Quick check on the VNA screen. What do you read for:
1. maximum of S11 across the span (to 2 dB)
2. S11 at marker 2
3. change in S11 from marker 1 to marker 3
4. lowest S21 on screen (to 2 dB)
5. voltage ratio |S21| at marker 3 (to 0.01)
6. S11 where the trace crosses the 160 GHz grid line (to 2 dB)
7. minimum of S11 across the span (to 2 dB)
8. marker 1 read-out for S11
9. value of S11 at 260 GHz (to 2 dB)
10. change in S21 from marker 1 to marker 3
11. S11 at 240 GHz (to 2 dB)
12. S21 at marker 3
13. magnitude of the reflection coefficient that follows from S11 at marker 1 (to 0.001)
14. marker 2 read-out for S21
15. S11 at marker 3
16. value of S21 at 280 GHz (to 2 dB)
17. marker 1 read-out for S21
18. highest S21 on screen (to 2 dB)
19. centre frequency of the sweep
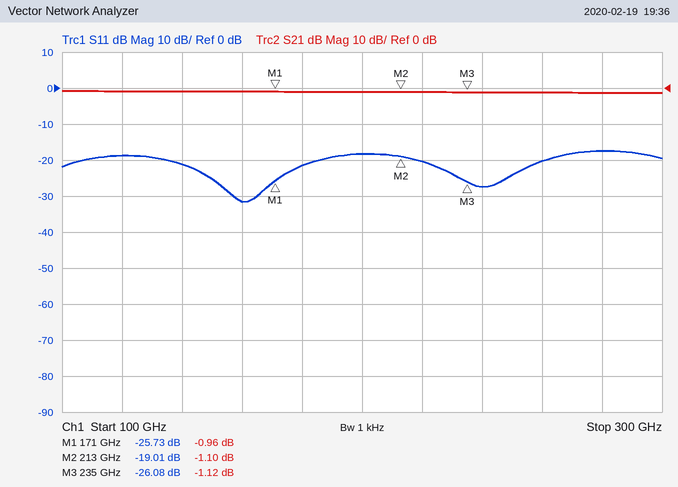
-18 dB
-19.01 dB
-0.35 dB
-2 dB
0.88
-32 dB
-32 dB
-25.73 dB
-20 dB
-0.16 dB
-28 dB
-1.12 dB
0.052
-1.10 dB
-26.08 dB
-2 dB
-0.96 dB
0 dB
200 GHz
